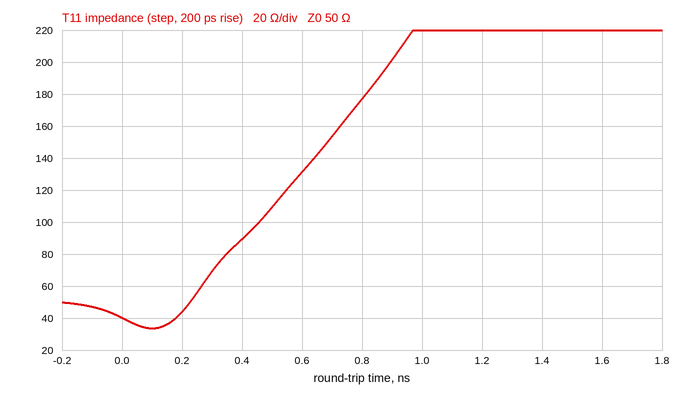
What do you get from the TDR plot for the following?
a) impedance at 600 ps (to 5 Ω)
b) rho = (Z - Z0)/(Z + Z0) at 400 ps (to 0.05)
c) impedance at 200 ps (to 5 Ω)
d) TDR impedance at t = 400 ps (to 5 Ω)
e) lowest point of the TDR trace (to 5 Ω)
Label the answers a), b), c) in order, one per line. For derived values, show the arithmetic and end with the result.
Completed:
a) 130 Ω
b) (90 − 50)/(90 + 50) ≈ +0.286, so +0.30 to the nearest 0.05
c) 45 Ω
d) 90 Ω
e) 35 Ω
